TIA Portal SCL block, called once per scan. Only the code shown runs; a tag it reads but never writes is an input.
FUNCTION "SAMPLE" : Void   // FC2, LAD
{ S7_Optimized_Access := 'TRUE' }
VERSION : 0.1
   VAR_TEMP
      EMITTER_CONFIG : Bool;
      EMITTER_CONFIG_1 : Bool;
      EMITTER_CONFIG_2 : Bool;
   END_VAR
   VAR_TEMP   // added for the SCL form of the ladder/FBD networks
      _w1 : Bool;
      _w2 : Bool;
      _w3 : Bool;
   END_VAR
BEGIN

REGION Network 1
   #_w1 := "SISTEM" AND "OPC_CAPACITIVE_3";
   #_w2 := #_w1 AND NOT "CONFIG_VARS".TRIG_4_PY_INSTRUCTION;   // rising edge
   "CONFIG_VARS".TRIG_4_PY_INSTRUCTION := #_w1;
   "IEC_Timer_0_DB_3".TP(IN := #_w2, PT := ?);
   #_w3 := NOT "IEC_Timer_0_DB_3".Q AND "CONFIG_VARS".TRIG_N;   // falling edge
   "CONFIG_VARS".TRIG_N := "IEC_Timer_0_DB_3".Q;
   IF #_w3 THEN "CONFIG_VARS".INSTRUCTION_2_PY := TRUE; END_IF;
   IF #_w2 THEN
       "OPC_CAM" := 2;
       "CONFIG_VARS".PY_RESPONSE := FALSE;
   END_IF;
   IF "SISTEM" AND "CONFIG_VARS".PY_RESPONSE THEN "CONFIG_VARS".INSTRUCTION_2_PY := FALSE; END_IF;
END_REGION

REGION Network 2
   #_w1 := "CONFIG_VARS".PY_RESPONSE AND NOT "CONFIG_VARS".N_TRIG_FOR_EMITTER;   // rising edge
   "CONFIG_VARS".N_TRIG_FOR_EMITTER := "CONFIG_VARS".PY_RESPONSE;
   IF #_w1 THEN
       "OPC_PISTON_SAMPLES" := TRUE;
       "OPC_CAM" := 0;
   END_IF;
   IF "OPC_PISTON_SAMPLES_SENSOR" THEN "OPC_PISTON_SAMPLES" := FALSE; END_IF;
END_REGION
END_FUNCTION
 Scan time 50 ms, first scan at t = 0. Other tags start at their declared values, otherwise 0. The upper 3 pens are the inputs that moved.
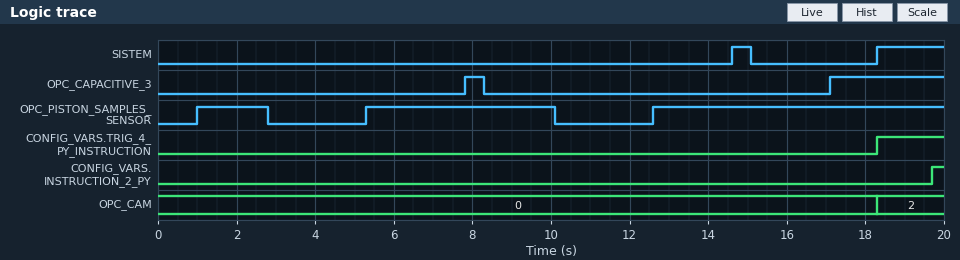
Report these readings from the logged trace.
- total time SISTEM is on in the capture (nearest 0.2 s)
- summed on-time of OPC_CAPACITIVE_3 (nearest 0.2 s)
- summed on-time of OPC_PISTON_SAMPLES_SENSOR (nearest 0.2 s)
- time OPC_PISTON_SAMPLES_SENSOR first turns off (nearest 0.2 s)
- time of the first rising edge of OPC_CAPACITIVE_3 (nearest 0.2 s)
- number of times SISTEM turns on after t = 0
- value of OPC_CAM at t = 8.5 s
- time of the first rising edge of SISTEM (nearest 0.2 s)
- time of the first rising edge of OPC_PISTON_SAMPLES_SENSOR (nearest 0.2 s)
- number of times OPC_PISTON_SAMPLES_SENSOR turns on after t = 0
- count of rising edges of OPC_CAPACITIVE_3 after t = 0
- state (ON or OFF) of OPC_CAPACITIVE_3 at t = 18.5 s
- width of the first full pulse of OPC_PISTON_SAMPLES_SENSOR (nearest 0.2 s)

2.2 s
3.4 s
14.0 s
2.8 s
7.8 s
2
0
14.6 s
1.0 s
3
2
ON
1.8 s
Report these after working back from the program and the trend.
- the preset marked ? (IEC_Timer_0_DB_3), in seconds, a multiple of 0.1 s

1.4 s
